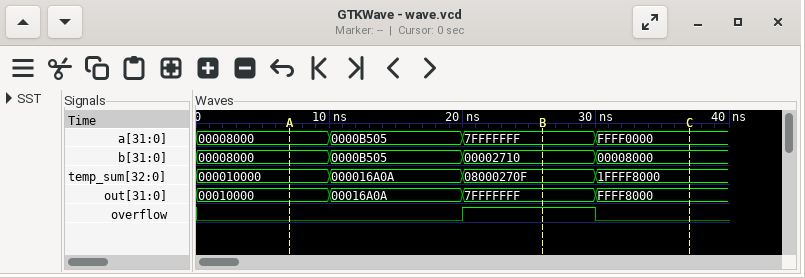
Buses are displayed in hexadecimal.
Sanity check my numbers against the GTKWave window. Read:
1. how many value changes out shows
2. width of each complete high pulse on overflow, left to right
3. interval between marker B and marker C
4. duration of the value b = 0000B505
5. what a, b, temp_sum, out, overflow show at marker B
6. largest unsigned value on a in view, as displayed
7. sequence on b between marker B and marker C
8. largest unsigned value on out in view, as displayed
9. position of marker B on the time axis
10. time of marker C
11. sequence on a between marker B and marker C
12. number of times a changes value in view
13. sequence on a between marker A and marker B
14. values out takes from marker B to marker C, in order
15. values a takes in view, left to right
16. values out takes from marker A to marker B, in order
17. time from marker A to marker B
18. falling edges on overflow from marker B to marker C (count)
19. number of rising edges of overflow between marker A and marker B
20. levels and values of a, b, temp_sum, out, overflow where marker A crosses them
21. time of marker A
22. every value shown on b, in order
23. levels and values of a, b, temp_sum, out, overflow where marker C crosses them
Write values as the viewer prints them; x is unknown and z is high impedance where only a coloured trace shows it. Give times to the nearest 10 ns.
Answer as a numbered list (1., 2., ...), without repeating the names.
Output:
1. 3
2. 10 ns
3. 10 ns
4. 10 ns
5. a=7FFFFFFF, b=00002710, temp_sum=08000270F, out=7FFFFFFF, overflow=1
6. FFFF0000
7. 00002710, 00008000
8. FFFF8000
9. 30 ns
10. 40 ns
11. 7FFFFFFF, FFFF0000
12. 3
13. 00008000, 0000B505, 7FFFFFFF
14. 7FFFFFFF, FFFF8000
15. 00008000, 0000B505, 7FFFFFFF, FFFF0000
16. 00010000, 00016A0A, 7FFFFFFF
17. 20 ns
18. 1
19. 1
20. a=00008000, b=00008000, temp_sum=000010000, out=00010000, overflow=0
21. 10 ns
22. 00008000, 0000B505, 00002710, 00008000
23. a=FFFF0000, b=00008000, temp_sum=1FFFF8000, out=FFFF8000, overflow=0
